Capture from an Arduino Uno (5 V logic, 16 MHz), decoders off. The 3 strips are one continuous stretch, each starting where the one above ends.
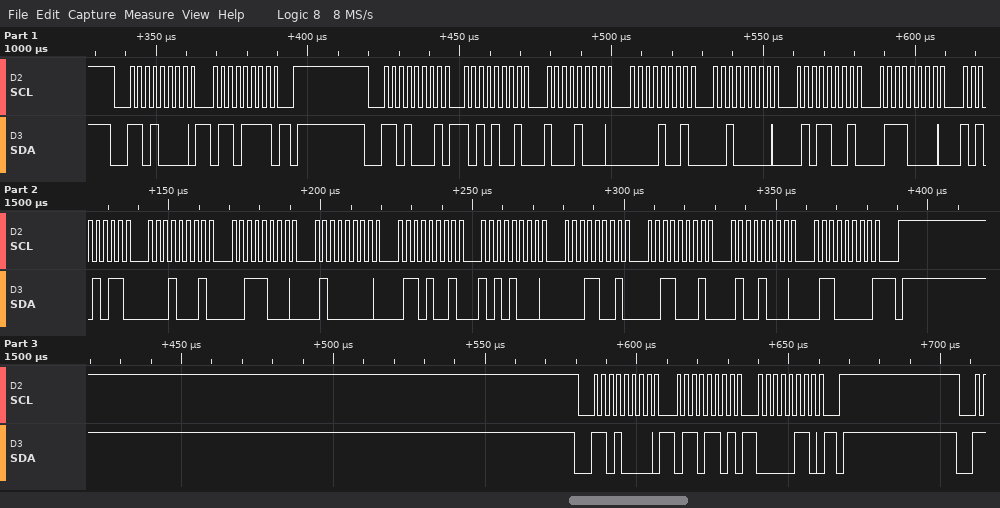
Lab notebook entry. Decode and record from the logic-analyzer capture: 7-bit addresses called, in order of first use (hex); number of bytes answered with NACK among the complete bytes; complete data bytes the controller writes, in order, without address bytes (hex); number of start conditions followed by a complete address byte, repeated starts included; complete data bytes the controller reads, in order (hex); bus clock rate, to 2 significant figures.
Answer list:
0x68
1
6F 6D 06
3
A9 88 09 20 59 70 AB 11 38 40 69 A8 19 31 48 60
400 kHz
